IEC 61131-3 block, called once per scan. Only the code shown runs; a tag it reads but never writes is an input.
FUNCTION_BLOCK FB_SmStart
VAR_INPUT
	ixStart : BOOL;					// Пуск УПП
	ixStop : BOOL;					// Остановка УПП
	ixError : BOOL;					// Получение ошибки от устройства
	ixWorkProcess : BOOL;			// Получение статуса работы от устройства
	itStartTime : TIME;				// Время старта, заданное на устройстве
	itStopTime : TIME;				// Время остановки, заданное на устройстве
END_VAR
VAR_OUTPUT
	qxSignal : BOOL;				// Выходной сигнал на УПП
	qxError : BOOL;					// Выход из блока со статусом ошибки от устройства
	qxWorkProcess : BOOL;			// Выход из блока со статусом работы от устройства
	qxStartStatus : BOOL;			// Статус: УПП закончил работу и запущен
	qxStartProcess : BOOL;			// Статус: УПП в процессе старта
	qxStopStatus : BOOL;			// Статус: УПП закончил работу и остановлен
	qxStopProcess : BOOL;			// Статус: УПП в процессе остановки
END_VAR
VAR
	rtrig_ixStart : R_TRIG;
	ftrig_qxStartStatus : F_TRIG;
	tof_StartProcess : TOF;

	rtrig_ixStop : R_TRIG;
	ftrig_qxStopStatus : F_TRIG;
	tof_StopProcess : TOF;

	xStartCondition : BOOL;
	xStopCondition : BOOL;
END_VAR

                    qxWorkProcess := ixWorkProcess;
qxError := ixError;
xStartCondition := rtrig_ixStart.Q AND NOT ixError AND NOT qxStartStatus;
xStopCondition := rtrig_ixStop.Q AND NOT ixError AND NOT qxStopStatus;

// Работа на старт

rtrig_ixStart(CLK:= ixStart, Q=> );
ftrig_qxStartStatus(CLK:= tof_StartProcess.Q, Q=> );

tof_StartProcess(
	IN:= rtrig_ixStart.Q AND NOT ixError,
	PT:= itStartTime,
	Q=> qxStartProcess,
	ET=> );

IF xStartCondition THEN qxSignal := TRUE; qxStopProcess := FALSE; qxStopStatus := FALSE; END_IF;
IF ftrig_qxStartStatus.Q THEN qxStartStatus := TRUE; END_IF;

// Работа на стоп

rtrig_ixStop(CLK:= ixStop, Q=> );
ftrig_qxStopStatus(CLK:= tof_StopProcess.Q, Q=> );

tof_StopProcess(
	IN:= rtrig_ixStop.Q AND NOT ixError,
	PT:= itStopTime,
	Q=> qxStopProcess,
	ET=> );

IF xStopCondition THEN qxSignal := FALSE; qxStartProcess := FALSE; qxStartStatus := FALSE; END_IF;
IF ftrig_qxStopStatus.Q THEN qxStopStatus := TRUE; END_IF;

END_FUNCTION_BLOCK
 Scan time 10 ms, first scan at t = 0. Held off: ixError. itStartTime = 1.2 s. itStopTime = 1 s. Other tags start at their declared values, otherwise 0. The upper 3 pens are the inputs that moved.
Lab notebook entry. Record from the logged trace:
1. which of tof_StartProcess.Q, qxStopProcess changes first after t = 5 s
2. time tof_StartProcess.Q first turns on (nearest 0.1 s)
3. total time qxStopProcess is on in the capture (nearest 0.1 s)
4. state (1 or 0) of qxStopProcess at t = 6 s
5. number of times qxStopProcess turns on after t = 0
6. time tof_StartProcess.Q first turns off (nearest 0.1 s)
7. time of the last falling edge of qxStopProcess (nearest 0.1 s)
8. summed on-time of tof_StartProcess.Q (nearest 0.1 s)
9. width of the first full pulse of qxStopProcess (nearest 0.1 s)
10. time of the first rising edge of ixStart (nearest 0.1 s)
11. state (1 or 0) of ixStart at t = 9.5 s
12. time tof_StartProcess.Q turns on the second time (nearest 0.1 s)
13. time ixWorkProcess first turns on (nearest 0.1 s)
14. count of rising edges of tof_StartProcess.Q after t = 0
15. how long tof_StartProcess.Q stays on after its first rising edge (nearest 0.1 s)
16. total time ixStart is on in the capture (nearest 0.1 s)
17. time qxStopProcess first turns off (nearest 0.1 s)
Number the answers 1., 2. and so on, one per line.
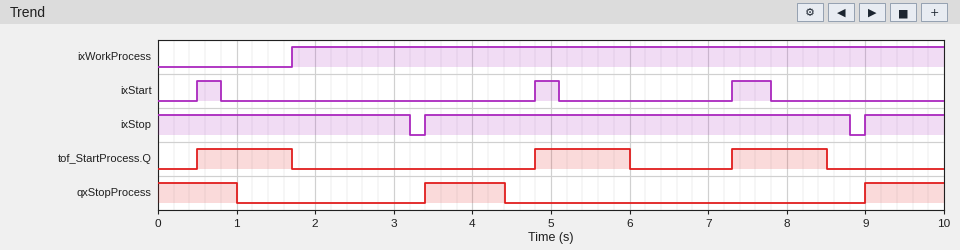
1. tof_StartProcess.Q
2. 0.5 s
3. 3.0 s
4. 0
5. 2
6. 1.7 s
7. 4.4 s
8. 3.6 s
9. 1.0 s
10. 0.5 s
11. 0
12. 4.8 s
13. 1.7 s
14. 3
15. 1.2 s
16. 1.1 s
17. 1.0 s
